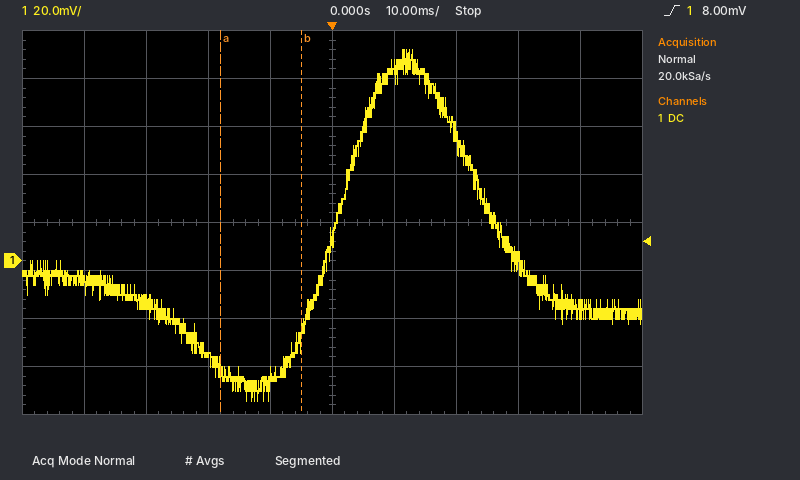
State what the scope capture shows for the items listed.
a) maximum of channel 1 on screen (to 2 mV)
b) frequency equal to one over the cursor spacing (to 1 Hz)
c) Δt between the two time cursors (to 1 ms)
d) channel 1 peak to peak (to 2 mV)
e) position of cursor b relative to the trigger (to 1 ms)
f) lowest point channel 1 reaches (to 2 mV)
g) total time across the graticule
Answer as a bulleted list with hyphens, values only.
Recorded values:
- 88 mV
- 77 Hz
- 13 ms
- 146 mV
- -5 ms
- -58 mV
- 100 ms
